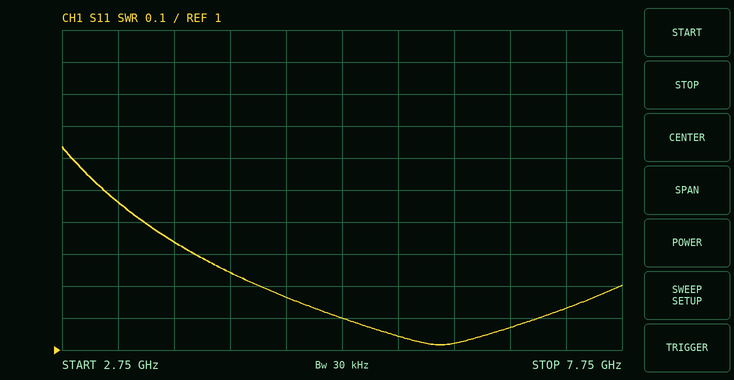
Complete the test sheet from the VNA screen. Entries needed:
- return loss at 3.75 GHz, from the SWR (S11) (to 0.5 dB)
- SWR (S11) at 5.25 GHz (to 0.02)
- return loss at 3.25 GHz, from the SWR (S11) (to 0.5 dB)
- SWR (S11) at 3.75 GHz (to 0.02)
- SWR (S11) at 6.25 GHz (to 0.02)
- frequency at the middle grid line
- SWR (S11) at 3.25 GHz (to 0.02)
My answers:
17.0 dB
1.10
14.5 dB
1.34
1.02
5.25 GHz
1.46
